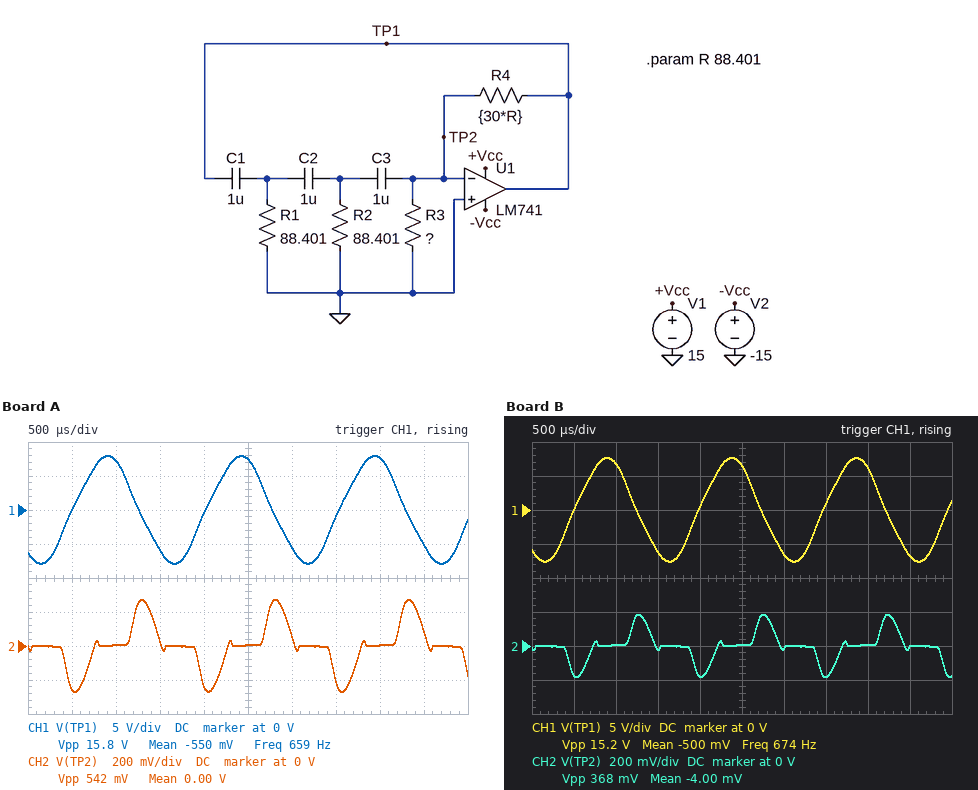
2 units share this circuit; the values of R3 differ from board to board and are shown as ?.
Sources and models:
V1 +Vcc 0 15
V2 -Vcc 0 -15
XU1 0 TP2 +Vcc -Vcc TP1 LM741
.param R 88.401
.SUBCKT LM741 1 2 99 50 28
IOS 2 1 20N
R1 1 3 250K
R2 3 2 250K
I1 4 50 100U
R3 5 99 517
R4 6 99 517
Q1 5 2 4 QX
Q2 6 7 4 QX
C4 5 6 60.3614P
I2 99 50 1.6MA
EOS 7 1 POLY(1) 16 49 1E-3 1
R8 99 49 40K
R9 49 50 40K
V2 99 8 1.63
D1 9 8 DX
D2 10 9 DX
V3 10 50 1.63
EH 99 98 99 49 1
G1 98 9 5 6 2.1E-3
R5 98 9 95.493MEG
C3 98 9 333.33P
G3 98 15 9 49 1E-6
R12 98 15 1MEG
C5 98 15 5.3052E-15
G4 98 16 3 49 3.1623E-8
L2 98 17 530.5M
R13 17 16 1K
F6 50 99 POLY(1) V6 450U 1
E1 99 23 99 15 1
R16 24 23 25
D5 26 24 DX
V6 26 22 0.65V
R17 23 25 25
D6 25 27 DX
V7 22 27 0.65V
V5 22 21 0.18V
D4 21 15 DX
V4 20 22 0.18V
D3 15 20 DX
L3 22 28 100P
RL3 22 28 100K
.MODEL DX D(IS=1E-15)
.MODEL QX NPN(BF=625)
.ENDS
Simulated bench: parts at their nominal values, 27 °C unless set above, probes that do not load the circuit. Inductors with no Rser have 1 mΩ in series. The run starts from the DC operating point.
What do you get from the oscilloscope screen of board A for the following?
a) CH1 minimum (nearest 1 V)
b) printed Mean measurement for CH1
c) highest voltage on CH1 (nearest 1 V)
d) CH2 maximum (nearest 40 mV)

-8 V
-550 mV
8 V
280 mV
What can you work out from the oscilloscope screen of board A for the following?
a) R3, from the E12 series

220 Ω
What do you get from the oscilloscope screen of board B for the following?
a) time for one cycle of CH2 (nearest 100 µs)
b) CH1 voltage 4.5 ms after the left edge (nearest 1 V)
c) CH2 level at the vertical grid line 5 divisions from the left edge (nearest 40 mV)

1.5 ms
-7 V
0 V
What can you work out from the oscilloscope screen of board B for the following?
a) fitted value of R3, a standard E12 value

120 Ω
